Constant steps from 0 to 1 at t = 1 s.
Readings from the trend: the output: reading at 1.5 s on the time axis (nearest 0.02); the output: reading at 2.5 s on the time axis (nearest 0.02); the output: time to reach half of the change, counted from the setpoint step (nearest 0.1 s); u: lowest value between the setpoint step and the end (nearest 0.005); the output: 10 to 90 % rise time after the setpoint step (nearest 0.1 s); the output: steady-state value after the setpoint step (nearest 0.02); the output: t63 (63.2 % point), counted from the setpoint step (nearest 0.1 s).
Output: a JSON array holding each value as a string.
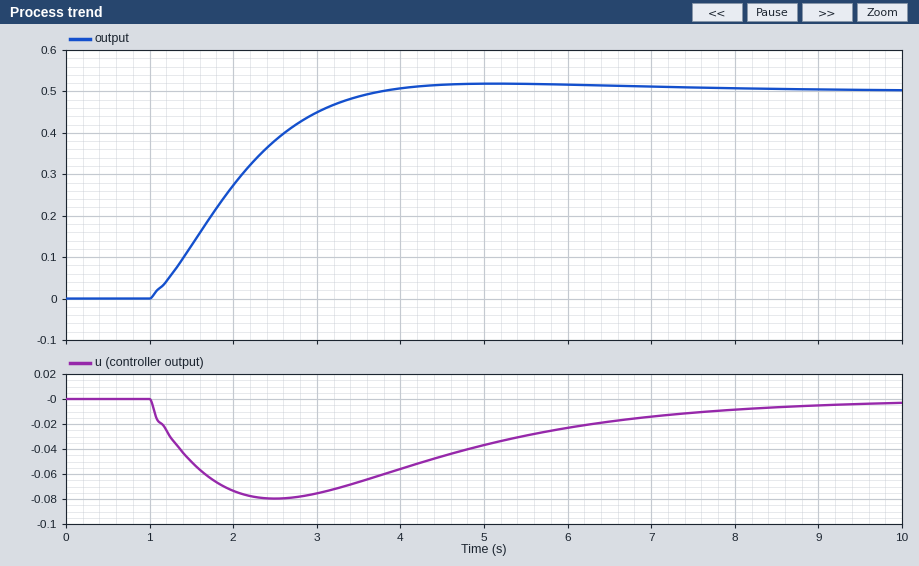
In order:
["0.12", "0.38", "0.9 s", "-0.080", "1.8 s", "0.50", "1.2 s"]
